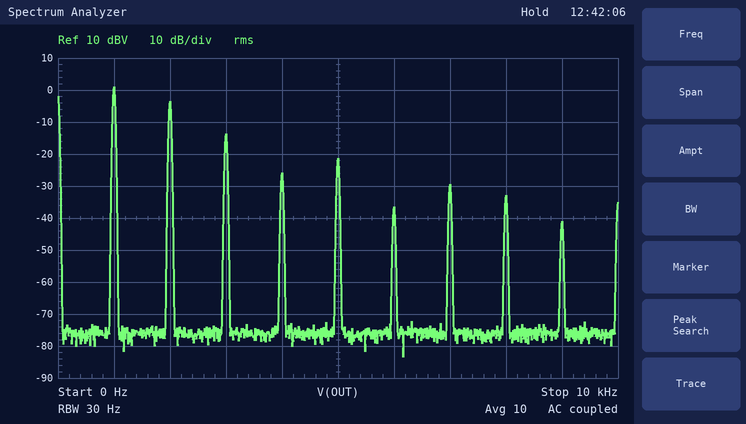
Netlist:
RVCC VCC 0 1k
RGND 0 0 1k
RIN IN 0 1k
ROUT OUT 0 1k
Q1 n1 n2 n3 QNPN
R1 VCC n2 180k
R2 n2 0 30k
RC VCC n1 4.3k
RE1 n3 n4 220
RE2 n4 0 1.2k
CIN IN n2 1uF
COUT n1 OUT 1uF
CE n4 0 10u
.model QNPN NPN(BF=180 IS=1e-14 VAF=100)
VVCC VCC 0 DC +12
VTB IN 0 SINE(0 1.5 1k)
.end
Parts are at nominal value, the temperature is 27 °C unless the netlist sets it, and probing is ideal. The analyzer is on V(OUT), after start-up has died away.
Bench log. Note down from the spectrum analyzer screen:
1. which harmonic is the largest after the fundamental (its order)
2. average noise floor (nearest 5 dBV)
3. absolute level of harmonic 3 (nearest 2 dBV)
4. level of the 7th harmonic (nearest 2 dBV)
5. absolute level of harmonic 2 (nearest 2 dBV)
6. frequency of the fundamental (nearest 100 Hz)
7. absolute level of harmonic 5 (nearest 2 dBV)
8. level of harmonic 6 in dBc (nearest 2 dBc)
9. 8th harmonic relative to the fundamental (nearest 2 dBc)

2
-75 dBV
-14 dBV
-30 dBV
-4 dBV
1.0 kHz
-22 dBV
-38 dBc
-34 dBc
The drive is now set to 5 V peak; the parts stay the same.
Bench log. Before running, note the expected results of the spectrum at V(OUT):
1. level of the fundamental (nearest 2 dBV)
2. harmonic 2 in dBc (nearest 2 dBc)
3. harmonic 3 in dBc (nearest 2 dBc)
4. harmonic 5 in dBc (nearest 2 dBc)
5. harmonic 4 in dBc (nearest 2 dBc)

2 dBV
-2 dBc
-6 dBc
-36 dBc
-14 dBc
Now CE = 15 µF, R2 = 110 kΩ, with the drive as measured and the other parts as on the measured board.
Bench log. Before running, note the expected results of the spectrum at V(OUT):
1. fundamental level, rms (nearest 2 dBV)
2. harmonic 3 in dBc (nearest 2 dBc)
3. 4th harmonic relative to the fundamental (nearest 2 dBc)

2 dBV
-22 dBc
-20 dBc
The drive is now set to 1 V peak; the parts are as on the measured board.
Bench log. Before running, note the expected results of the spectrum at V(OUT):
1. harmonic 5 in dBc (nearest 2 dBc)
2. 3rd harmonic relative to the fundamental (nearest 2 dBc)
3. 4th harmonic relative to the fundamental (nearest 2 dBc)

-26 dBc
-20 dBc
-22 dBc
